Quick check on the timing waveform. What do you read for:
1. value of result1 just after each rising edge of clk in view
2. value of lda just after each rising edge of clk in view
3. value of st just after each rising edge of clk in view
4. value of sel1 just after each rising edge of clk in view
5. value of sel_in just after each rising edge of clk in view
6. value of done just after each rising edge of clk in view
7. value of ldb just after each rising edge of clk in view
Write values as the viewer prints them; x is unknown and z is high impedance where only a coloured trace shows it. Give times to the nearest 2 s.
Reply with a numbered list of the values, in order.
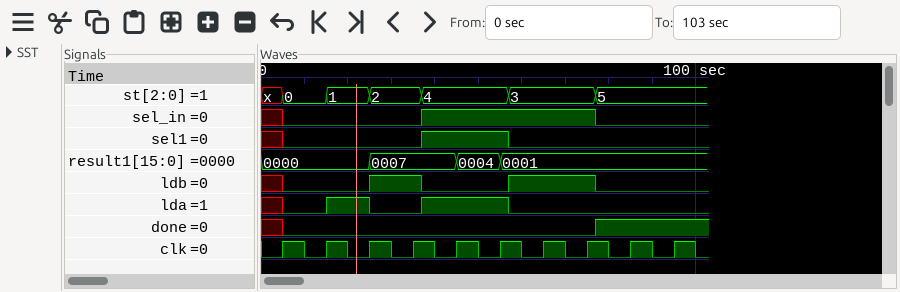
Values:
1. 0000, 0000, 0007, 0007, 0004, 0001, 0001, 0001, 0001, 0001
2. 0 1 0 0 1 1 0 0 0 0
3. 0, 1, 2, 2, 4, 4, 3, 3, 5, 5
4. 0 0 0 0 1 1 0 0 0 0
5. 0 0 0 0 1 1 1 1 0 0
6. 0 0 0 0 0 0 0 0 1 1
7. 0 0 1 1 0 0 1 1 0 0
